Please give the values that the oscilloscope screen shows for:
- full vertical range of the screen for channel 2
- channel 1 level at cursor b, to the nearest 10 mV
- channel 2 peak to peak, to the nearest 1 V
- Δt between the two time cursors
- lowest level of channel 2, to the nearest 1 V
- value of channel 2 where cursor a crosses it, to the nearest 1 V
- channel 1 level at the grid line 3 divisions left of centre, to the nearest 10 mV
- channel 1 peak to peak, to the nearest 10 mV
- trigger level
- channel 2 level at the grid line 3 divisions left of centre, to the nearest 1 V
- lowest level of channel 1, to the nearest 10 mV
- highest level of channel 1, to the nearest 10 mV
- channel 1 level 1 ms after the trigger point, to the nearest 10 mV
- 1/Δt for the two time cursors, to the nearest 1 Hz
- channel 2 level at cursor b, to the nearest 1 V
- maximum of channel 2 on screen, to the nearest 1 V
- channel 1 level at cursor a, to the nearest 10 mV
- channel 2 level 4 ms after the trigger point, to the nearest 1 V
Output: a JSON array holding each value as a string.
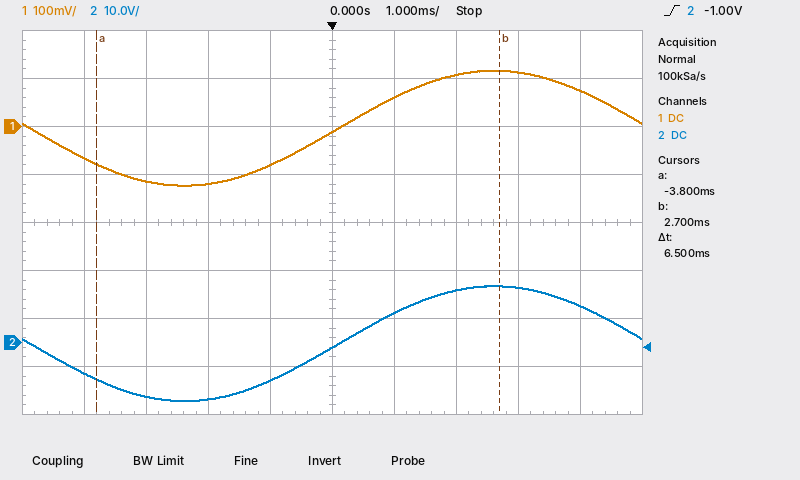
["80 V", "120 mV", "24 V", "6.5 ms", "-12 V", "-8 V", "-110 mV", "240 mV", "-1.00 V", "-11 V", "-120 mV", "120 mV", "60 mV", "154 Hz", "12 V", "12 V", "-80 mV", "8 V"]
